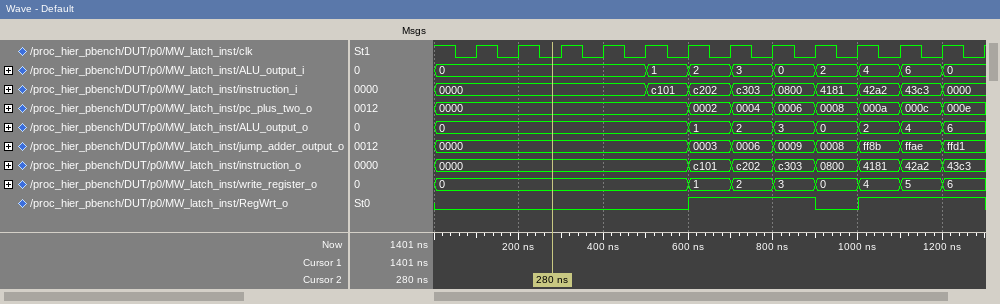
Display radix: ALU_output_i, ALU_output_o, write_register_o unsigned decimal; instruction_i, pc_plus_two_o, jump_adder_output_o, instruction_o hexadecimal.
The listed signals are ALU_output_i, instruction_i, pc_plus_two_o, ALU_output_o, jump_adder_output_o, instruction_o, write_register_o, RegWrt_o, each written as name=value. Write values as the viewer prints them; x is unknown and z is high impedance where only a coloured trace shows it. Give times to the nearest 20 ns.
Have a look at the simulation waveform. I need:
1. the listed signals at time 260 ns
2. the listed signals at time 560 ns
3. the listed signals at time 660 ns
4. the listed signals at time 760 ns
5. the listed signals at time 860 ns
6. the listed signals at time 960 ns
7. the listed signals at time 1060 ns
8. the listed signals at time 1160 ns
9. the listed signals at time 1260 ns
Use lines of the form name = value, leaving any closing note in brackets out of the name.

the listed signals at time 260 ns = ALU_output_i=0, instruction_i=0000, pc_plus_two_o=0000, ALU_output_o=0, jump_adder_output_o=0000, instruction_o=0000, write_register_o=0, RegWrt_o=0
the listed signals at time 560 ns = ALU_output_i=1, instruction_i=c101, pc_plus_two_o=0000, ALU_output_o=0, jump_adder_output_o=0000, instruction_o=0000, write_register_o=0, RegWrt_o=0
the listed signals at time 660 ns = ALU_output_i=2, instruction_i=c202, pc_plus_two_o=0002, ALU_output_o=1, jump_adder_output_o=0003, instruction_o=c101, write_register_o=1, RegWrt_o=1
the listed signals at time 760 ns = ALU_output_i=3, instruction_i=c303, pc_plus_two_o=0004, ALU_output_o=2, jump_adder_output_o=0006, instruction_o=c202, write_register_o=2, RegWrt_o=1
the listed signals at time 860 ns = ALU_output_i=0, instruction_i=0800, pc_plus_two_o=0006, ALU_output_o=3, jump_adder_output_o=0009, instruction_o=c303, write_register_o=3, RegWrt_o=1
the listed signals at time 960 ns = ALU_output_i=2, instruction_i=4181, pc_plus_two_o=0008, ALU_output_o=0, jump_adder_output_o=0008, instruction_o=0800, write_register_o=0, RegWrt_o=0
the listed signals at time 1060 ns = ALU_output_i=4, instruction_i=42a2, pc_plus_two_o=000a, ALU_output_o=2, jump_adder_output_o=ff8b, instruction_o=4181, write_register_o=4, RegWrt_o=1
the listed signals at time 1160 ns = ALU_output_i=6, instruction_i=43c3, pc_plus_two_o=000c, ALU_output_o=4, jump_adder_output_o=ffae, instruction_o=42a2, write_register_o=5, RegWrt_o=1
the listed signals at time 1260 ns = ALU_output_i=0, instruction_i=0000, pc_plus_two_o=000e, ALU_output_o=6, jump_adder_output_o=ffd1, instruction_o=43c3, write_register_o=6, RegWrt_o=1
